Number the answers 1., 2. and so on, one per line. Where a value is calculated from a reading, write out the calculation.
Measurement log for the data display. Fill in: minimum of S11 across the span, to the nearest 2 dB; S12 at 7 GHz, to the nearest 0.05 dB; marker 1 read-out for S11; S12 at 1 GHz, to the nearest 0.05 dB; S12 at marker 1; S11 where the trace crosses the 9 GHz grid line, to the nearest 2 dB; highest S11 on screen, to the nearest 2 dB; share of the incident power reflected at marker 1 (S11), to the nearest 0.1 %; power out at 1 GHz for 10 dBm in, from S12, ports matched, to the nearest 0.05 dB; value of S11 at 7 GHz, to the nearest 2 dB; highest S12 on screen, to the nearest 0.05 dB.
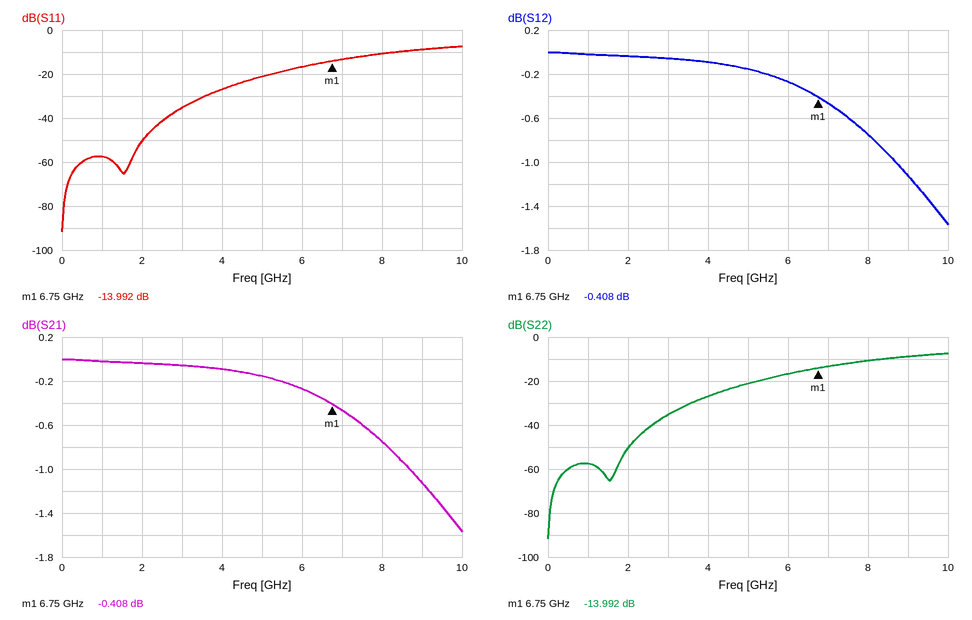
1. -92 dB
2. -0.45 dB
3. -13.992 dB
4. 0.00 dB
5. -0.408 dB
6. -8 dB
7. -8 dB
8. 10^(-13.992/10) ≈ 4.0 %
9. 10 dBm + (0.00 dB) = 10.00 dBm
10. -14 dB
11. 0.00 dB
